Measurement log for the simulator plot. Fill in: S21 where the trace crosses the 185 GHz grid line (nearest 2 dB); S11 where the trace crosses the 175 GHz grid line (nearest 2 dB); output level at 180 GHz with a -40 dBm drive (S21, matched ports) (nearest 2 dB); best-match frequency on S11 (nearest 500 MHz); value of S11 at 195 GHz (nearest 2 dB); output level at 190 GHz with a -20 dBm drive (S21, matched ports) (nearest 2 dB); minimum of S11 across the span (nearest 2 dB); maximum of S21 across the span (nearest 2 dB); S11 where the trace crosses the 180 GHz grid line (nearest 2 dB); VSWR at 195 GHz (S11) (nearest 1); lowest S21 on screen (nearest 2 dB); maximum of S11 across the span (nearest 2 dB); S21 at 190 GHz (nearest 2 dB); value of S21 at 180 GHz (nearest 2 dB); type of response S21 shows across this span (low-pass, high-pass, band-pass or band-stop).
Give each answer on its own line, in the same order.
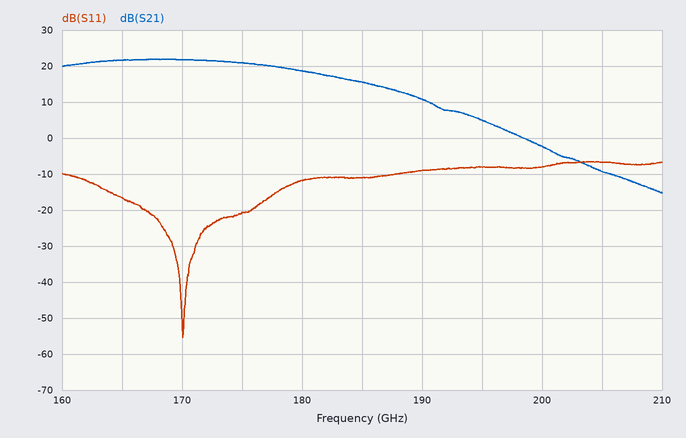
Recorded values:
16 dB
-20 dB
-22 dBm
170.0 GHz
-8 dB
-10 dBm
-56 dB
22 dB
-12 dB
2
-16 dB
-6 dB
10 dB
18 dB
low-pass
